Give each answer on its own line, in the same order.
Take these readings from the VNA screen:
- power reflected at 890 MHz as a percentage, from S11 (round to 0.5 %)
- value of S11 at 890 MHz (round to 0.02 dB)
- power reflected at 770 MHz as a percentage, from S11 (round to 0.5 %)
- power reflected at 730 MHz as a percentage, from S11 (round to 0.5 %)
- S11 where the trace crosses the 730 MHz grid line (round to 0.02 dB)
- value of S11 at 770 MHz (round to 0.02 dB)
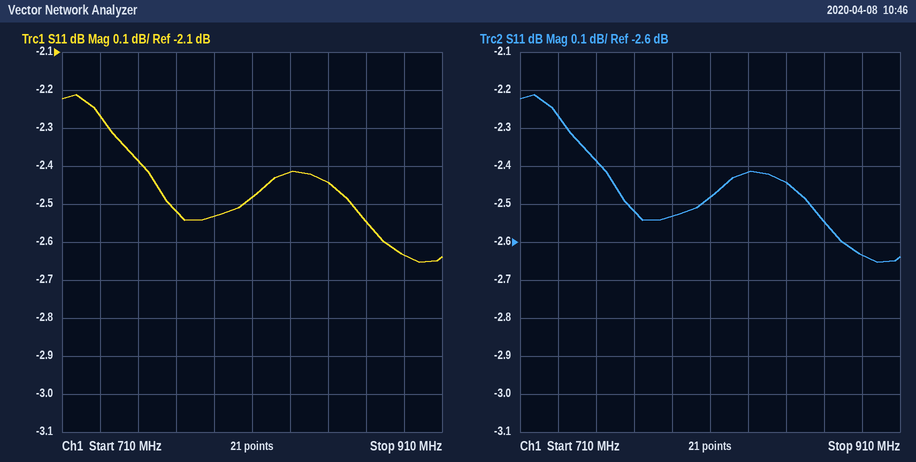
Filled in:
54.5 %
-2.64 dB
56.0 %
59.5 %
-2.26 dB
-2.52 dB
